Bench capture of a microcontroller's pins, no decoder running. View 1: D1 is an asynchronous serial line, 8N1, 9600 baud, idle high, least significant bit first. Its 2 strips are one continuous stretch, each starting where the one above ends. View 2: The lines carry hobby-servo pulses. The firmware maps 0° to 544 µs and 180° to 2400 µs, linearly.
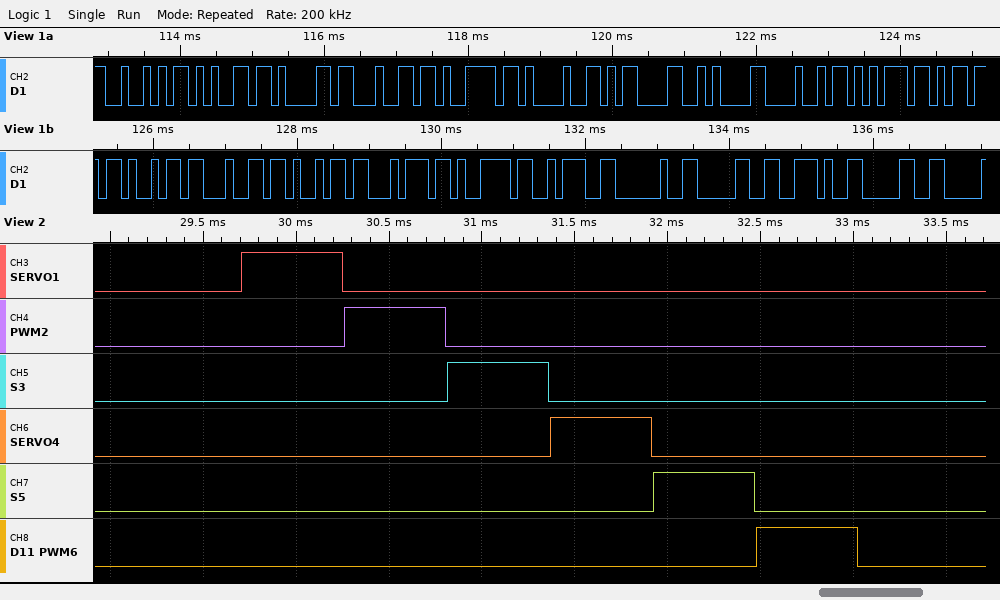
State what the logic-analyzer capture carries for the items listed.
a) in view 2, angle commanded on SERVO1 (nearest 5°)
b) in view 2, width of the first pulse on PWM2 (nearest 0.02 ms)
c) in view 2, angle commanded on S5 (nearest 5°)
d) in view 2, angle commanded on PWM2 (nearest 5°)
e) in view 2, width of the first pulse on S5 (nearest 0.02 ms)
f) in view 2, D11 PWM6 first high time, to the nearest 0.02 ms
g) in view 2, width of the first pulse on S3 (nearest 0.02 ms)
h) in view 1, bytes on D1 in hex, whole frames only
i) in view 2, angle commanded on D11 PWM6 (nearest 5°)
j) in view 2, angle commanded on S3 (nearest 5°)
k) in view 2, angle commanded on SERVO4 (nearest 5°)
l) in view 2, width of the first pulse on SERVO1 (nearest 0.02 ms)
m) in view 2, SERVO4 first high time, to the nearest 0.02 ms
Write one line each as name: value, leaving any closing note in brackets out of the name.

in view 2, angle commanded on SERVO1: 0°
in view 2, width of the first pulse on PWM2: 0.54 ms
in view 2, angle commanded on S5: 0°
in view 2, angle commanded on PWM2: 0°
in view 2, width of the first pulse on S5: 0.54 ms
in view 2, D11 PWM6 first high time, to the nearest 0.02 ms: 0.54 ms
in view 2, width of the first pulse on S3: 0.54 ms
in view 1, bytes on D1 in hex, whole frames only: 52 65 61 64 79 21 0D 0A 48 75 6D 69 64 69 74 79 3A 20 30 2E 30
in view 2, angle commanded on D11 PWM6: 0°
in view 2, angle commanded on S3: 0°
in view 2, angle commanded on SERVO4: 0°
in view 2, width of the first pulse on SERVO1: 0.54 ms
in view 2, SERVO4 first high time, to the nearest 0.02 ms: 0.54 ms
